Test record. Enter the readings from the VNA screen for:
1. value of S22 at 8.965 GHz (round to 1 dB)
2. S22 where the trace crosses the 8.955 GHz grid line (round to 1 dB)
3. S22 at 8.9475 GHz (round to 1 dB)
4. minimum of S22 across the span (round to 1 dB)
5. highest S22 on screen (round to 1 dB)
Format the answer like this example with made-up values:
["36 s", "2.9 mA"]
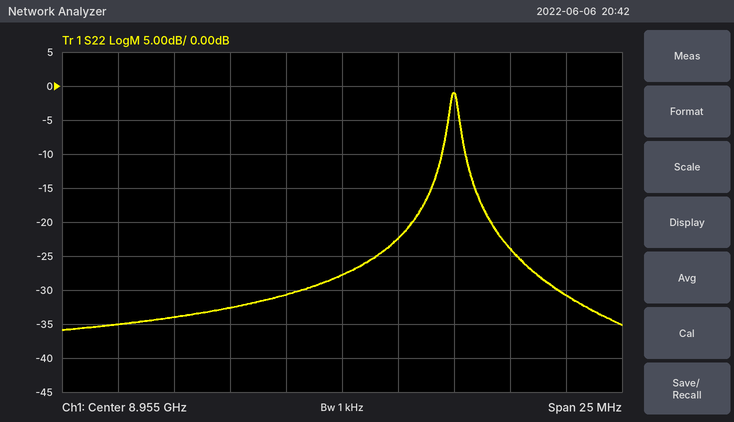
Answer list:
["-31 dB", "-28 dB", "-34 dB", "-36 dB", "-1 dB"]
